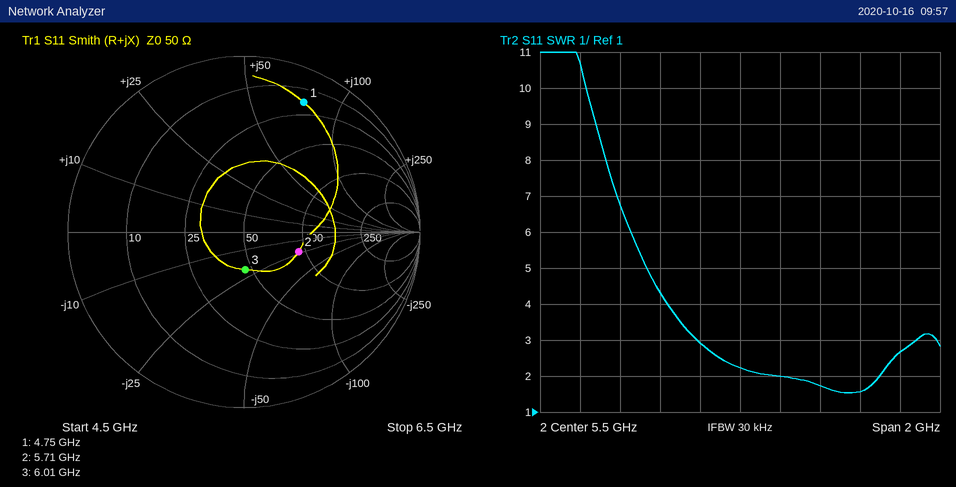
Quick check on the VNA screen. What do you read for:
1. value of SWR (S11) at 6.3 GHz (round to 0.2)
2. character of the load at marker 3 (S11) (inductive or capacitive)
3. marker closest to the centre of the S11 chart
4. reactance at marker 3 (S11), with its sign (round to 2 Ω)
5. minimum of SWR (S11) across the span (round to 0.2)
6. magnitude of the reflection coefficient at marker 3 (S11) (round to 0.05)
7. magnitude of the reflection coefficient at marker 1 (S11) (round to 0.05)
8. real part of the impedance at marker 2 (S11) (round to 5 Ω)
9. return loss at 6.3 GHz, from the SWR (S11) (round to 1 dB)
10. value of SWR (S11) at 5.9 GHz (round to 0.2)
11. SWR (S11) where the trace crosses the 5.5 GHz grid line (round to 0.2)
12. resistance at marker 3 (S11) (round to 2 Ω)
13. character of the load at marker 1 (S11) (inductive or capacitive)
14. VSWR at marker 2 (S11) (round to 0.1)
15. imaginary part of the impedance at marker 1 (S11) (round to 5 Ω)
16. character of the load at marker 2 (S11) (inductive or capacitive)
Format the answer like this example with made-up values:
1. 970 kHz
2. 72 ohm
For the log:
1. 2.6
2. capacitive
3. marker 3
4. -20 Ω
5. 1.6
6. 0.20
7. 0.80
8. 90 Ω
9. 7 dB
10. 1.8
11. 2.2
12. 46 Ω
13. inductive
14. 2.0
15. +75 Ω
16. capacitive
